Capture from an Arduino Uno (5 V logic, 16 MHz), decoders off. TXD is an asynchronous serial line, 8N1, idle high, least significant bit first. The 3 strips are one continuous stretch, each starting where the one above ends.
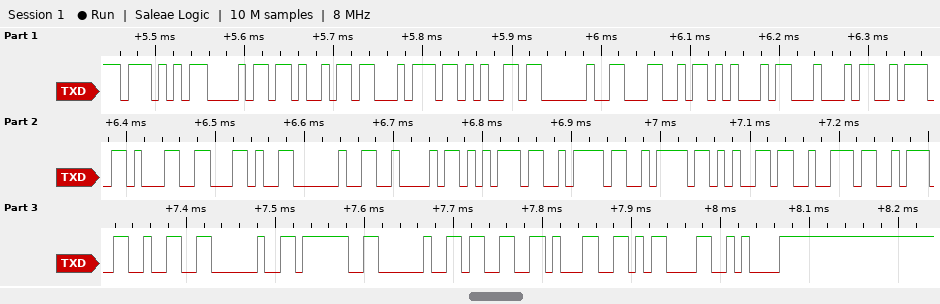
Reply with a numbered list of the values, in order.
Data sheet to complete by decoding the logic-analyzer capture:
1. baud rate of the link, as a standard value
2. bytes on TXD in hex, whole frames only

1. 115200 baud
2. 57 68 69 74 65 20 4C 45 44 3A 31 2C 20 42 75 7A 7A 65 72 3A 32 20 3F 20 33 31 0D 0A
